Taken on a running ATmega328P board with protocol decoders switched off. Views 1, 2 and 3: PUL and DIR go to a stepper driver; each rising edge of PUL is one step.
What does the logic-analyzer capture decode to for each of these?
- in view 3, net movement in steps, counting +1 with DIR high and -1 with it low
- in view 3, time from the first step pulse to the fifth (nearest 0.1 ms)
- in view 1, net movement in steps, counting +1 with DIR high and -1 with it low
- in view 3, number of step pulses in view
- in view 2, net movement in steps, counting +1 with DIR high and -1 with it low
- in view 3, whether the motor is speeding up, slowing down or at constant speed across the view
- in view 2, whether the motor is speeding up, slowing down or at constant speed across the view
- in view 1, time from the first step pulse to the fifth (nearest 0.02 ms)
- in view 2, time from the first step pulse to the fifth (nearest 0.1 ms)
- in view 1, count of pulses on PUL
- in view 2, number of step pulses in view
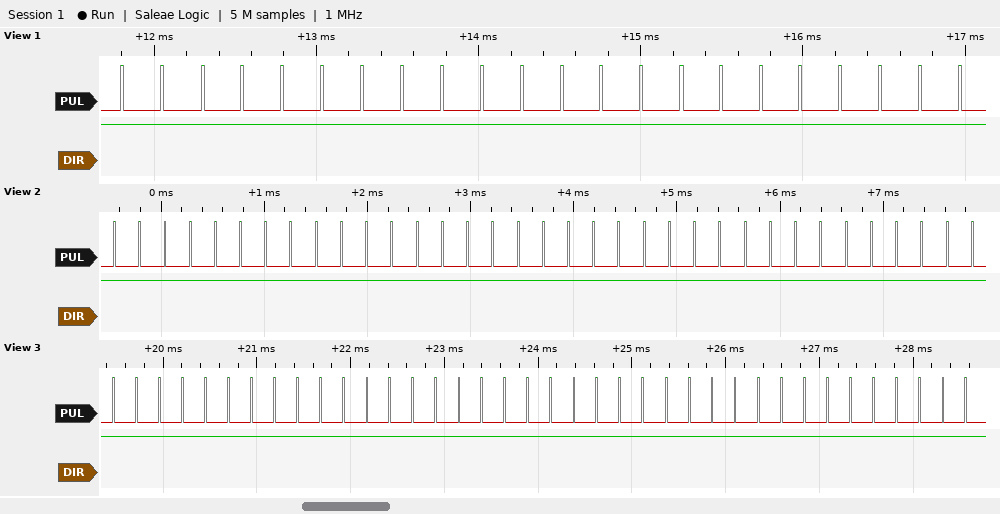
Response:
+38
1.0 ms
+22
38
+35
constant speed
constant speed
0.98 ms
1.0 ms
22
35
